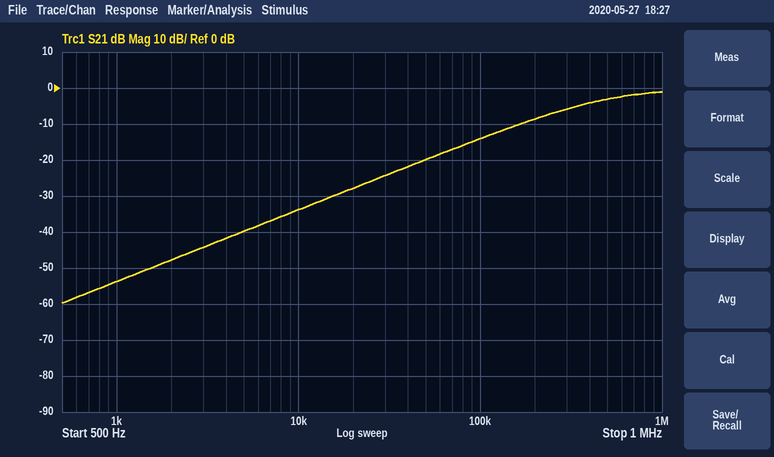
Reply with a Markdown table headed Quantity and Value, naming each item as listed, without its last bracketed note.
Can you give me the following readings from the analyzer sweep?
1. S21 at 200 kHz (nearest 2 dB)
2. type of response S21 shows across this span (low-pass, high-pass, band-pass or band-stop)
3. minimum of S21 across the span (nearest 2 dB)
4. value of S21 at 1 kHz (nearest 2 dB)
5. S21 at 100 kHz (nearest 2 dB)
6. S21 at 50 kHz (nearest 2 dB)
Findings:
| Quantity | Value |
|---|---|
| S21 at 200 kHz | -8 dB |
| type of response S21 shows across this span | high-pass |
| minimum of S21 across the span | -60 dB |
| value of S21 at 1 kHz | -54 dB |
| S21 at 100 kHz | -14 dB |
| S21 at 50 kHz | -20 dB |
